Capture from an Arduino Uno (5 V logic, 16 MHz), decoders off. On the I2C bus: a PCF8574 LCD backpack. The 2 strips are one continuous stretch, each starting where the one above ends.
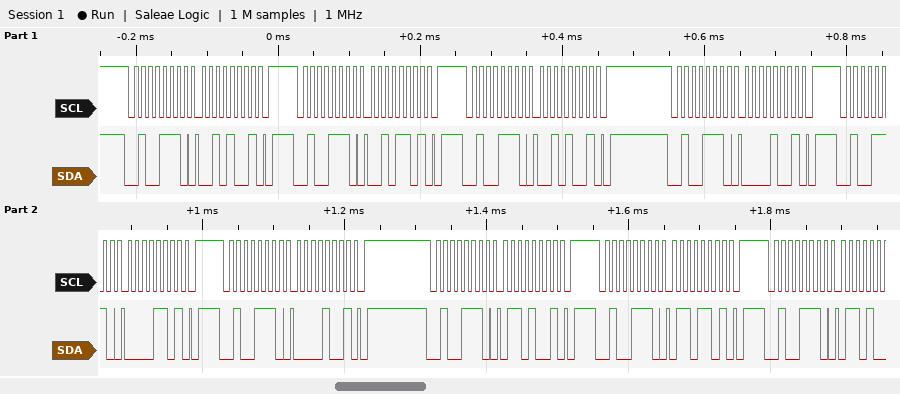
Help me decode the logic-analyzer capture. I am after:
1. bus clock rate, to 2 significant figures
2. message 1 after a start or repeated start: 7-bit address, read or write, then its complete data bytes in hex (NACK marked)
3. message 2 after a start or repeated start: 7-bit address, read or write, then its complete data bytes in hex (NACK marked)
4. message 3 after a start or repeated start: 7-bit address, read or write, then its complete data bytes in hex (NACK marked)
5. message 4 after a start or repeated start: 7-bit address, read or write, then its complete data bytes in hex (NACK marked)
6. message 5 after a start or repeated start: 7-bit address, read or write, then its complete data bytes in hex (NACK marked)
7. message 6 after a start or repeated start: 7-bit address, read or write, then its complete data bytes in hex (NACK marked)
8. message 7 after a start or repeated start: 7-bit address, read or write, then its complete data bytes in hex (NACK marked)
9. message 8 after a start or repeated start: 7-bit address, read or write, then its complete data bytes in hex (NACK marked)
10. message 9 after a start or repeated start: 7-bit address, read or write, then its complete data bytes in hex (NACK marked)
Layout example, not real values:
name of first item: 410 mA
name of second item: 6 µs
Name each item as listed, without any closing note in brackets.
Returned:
bus clock rate, to 2 significant figures: 100 kHz
message 1 after a start or repeated start: 7-bit address, read or write, then its complete data bytes in hex: 0x27 write: 29
message 2 after a start or repeated start: 7-bit address, read or write, then its complete data bytes in hex: 0x27 write: 2D
message 3 after a start or repeated start: 7-bit address, read or write, then its complete data bytes in hex: 0x27 write: 29
message 4 after a start or repeated start: 7-bit address, read or write, then its complete data bytes in hex: 0x27 write: 09
message 5 after a start or repeated start: 7-bit address, read or write, then its complete data bytes in hex: 0x27 write: 0D
message 6 after a start or repeated start: 7-bit address, read or write, then its complete data bytes in hex: 0x27 write: 09
message 7 after a start or repeated start: 7-bit address, read or write, then its complete data bytes in hex: 0x27 write: 69
message 8 after a start or repeated start: 7-bit address, read or write, then its complete data bytes in hex: 0x27 write: 6D
message 9 after a start or repeated start: 7-bit address, read or write, then its complete data bytes in hex: 0x27 write
